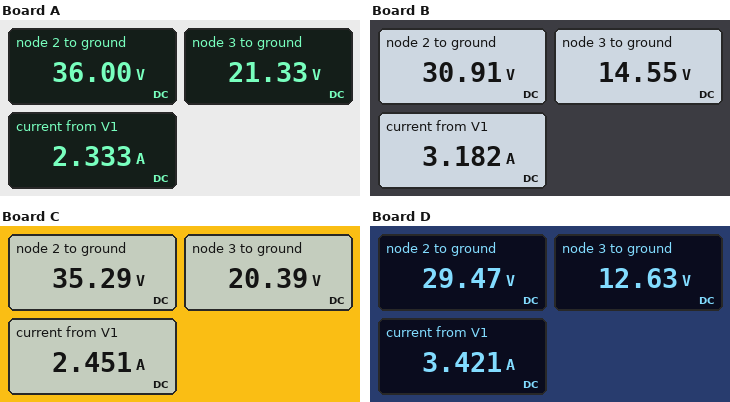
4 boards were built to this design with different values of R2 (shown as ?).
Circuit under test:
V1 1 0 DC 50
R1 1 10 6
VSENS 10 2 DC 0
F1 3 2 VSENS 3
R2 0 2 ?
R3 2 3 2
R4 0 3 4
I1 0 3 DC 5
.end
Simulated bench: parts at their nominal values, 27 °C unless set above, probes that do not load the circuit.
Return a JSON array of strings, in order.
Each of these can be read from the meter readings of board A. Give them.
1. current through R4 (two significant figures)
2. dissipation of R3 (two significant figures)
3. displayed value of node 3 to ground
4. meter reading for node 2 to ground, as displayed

["5.3 A", "110 W", "21.33 V", "36.00 V"]
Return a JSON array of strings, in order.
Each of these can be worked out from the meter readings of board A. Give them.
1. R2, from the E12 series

["18 Ω"]
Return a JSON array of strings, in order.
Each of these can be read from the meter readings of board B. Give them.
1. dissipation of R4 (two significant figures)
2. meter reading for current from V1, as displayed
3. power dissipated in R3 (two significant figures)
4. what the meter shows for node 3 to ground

["53 W", "3.182 A", "130 W", "14.55 V"]
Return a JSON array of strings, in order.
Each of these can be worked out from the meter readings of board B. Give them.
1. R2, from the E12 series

["6.8 Ω"]
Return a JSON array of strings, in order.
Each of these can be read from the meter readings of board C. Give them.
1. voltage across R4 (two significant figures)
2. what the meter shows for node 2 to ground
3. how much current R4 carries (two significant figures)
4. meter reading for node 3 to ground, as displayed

["20 V", "35.29 V", "5.1 A", "20.39 V"]
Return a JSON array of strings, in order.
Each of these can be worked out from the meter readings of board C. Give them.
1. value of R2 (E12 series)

["15 Ω"]
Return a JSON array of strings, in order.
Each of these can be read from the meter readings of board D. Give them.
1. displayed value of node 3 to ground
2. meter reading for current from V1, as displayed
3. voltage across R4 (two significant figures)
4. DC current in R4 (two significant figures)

["12.63 V", "3.421 A", "13 V", "3.2 A"]
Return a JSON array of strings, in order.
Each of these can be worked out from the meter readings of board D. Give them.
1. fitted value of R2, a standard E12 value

["5.6 Ω"]
